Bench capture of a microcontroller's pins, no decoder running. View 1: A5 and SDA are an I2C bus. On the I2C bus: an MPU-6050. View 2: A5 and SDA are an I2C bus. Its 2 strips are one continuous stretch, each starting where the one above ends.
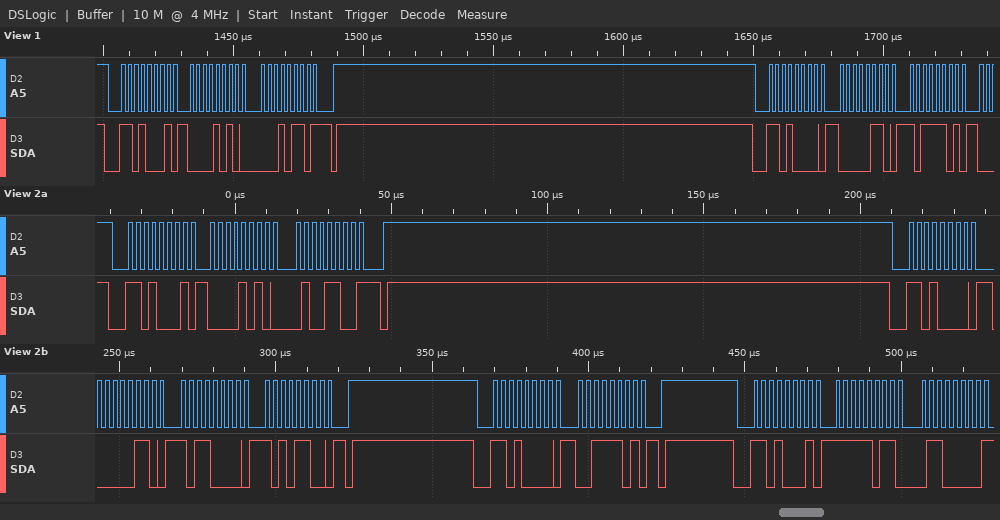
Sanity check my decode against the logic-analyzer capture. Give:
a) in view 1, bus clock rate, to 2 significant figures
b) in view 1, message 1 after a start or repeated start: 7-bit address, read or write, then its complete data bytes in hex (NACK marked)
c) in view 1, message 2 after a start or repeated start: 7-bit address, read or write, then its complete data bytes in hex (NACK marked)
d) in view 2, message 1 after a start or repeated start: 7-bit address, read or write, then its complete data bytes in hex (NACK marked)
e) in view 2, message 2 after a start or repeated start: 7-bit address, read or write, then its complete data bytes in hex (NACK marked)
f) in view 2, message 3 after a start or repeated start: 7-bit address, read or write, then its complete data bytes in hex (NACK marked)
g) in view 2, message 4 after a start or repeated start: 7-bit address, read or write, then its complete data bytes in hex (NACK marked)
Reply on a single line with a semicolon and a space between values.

400 kHz; 0x68 read: 0A 16 NACK; 0x68 write: 06 BD; 0x68 read: 0A 4C NACK; 0x68 write: 06 B0 AC; 0x68 write: 3D; 0x68 read: FB 60 NACK
